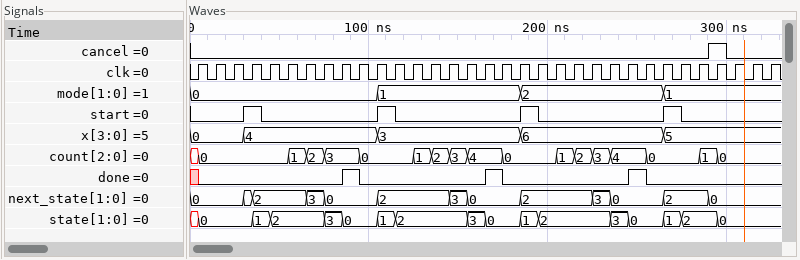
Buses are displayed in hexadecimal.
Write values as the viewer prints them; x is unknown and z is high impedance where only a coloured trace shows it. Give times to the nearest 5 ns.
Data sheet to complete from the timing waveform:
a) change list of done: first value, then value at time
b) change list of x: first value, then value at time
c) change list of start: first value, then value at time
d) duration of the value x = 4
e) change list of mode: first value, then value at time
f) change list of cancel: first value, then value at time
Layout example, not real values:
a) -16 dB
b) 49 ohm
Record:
a) x, 0 at 5 ns, 1 at 85 ns, 0 at 95 ns, 1 at 165 ns, 0 at 175 ns, 1 at 245 ns, 0 at 255 ns
b) 0, 4 at 30 ns, 3 at 105 ns, 6 at 185 ns, 5 at 265 ns
c) 0, 1 at 30 ns, 0 at 40 ns, 1 at 105 ns, 0 at 115 ns, 1 at 185 ns, 0 at 195 ns, 1 at 265 ns, 0 at 275 ns
d) 75 ns
e) 0, 1 at 105 ns, 2 at 185 ns, 1 at 265 ns
f) 0, 1 at 290 ns, 0 at 300 ns
